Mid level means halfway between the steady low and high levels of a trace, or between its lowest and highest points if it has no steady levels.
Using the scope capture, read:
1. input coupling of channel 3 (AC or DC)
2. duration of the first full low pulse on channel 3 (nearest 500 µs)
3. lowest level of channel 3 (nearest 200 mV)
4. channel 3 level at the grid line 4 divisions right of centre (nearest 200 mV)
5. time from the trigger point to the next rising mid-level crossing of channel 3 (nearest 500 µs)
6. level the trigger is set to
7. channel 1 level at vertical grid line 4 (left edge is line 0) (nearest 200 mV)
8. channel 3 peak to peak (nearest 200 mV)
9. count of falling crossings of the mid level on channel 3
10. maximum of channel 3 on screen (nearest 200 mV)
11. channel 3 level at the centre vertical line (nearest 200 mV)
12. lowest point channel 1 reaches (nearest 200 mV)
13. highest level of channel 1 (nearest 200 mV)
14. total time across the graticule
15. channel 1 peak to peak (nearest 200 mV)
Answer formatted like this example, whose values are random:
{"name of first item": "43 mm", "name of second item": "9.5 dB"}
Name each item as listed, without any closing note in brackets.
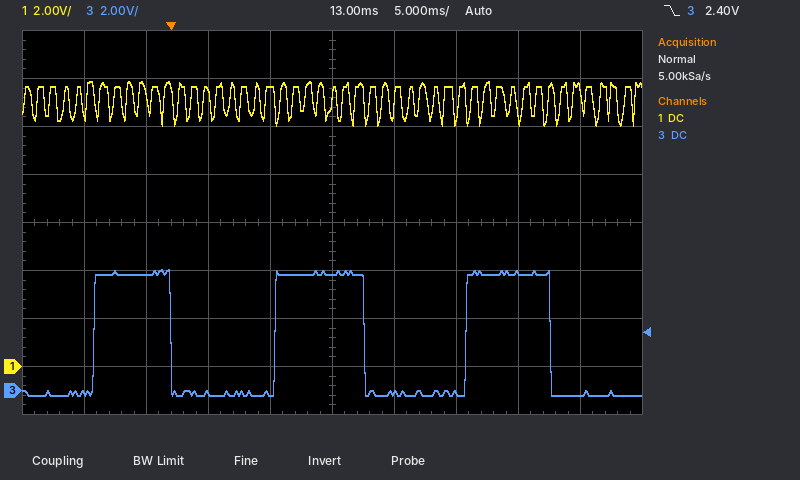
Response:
{"input coupling of channel 3": "DC", "duration of the first full low pulse on channel 3": "8.5 ms", "lowest level of channel 3": "-200 mV", "channel 3 level at the grid line 4 divisions right of centre": "-200 mV", "time from the trigger point to the next rising mid-level crossing of channel 3": "8.5 ms", "level the trigger is set to": "2.40 V", "channel 1 level at vertical grid line 4 (left edge is line 0)": "11.6 V", "channel 3 peak to peak": "5.2 V", "count of falling crossings of the mid level on channel 3": "3", "maximum of channel 3 on screen": "5.0 V", "channel 3 level at the centre vertical line": "4.8 V", "lowest point channel 1 reaches": "10.0 V", "highest level of channel 1": "11.8 V", "total time across the graticule": "50 ms", "channel 1 peak to peak": "1.8 V"}
